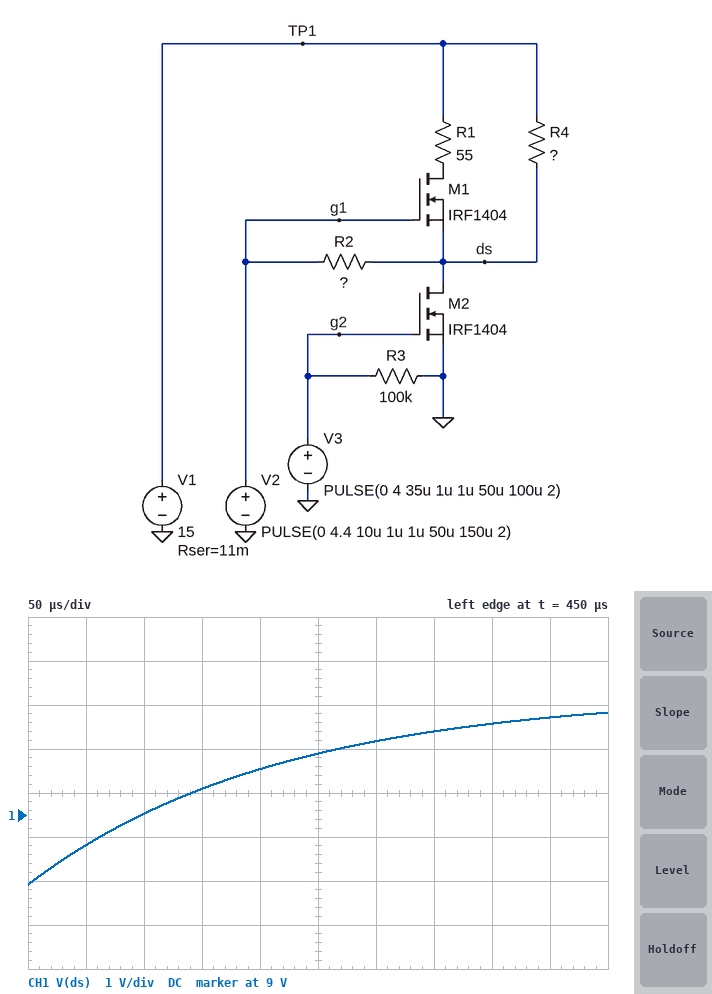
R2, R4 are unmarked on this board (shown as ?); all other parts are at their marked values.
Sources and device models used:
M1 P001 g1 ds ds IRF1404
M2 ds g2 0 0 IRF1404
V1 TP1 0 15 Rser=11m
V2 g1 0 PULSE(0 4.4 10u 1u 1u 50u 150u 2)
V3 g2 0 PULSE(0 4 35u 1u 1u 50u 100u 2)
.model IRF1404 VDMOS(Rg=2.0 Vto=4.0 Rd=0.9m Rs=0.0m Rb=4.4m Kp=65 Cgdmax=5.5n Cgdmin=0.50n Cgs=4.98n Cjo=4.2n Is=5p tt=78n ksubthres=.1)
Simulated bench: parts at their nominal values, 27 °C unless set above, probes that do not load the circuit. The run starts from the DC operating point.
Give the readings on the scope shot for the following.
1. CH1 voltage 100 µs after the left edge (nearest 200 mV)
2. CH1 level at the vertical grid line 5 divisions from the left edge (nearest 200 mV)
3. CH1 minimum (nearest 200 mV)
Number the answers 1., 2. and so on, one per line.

1. 9.0 V
2. 10.4 V
3. 7.4 V
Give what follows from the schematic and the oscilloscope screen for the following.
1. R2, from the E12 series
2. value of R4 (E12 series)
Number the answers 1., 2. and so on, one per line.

1. 120 kΩ
2. 33 kΩ
